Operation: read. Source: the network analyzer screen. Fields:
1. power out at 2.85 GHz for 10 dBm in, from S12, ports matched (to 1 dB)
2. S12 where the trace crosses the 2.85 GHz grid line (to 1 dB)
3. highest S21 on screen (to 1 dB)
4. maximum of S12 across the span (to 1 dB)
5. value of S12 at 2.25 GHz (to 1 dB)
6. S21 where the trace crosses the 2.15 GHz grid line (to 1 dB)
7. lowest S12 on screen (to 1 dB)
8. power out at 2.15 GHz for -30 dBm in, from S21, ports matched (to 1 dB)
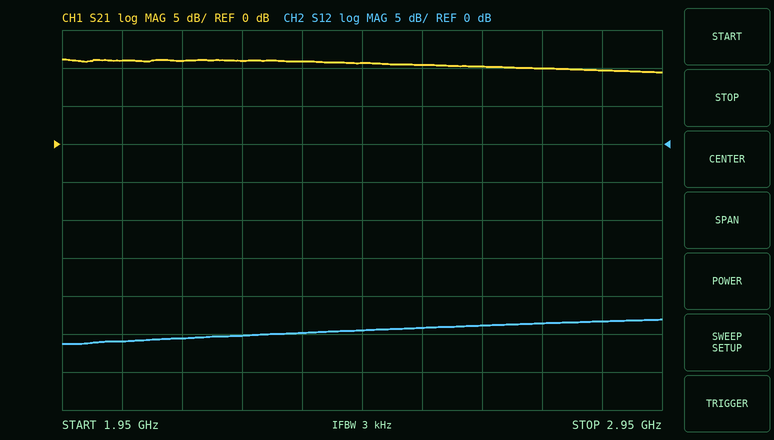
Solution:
-13 dBm
-23 dB
11 dB
-23 dB
-25 dB
11 dB
-26 dB
-19 dBm
